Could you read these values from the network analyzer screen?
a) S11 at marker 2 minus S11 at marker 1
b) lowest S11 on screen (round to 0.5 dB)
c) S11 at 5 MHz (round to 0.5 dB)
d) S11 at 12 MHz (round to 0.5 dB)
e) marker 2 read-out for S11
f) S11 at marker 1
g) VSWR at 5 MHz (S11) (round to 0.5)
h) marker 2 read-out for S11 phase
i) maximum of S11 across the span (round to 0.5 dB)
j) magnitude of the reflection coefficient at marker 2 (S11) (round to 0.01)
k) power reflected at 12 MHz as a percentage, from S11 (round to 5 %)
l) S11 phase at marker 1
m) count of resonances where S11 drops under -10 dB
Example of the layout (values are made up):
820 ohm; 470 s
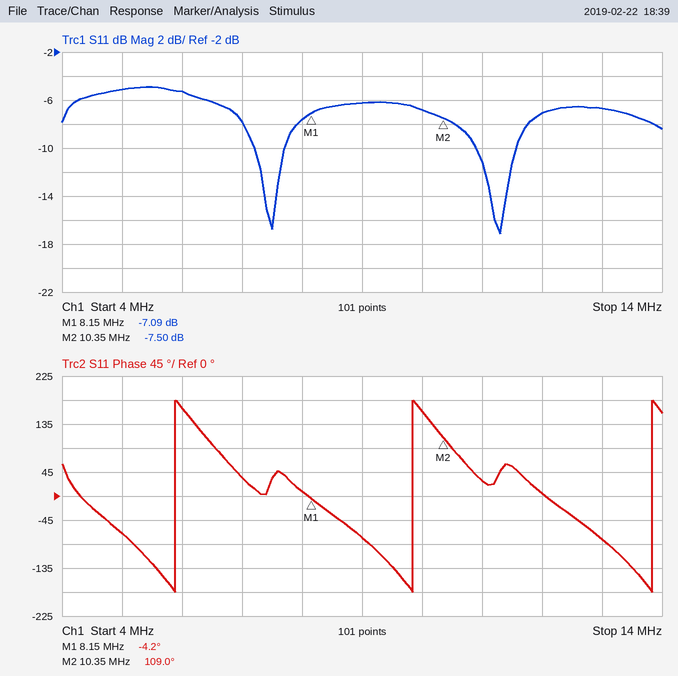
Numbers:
-0.41 dB; -17.0 dB; -5.0 dB; -7.0 dB; -7.50 dB; -7.09 dB; 3.5; 109.0°; -5.0 dB; 0.42; 20 %; -4.2°; 2
